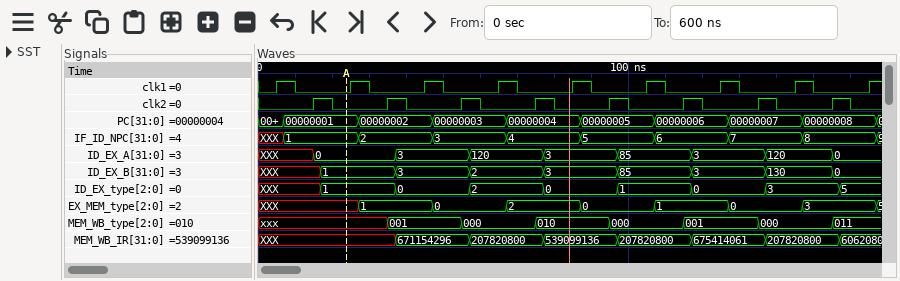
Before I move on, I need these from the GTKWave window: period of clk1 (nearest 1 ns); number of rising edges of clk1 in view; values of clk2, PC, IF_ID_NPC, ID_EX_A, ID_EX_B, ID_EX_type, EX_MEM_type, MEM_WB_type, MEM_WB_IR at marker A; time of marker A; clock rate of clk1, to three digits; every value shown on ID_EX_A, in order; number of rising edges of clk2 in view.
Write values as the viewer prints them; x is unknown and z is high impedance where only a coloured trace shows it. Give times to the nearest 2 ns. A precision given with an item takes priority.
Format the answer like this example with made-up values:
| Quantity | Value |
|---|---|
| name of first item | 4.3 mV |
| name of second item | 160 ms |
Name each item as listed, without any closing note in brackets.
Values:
| Quantity | Value |
|---|---|
| period of clk1 | 20 ns |
| number of rising edges of clk1 in view | 9 |
| values of clk2, PC, IF_ID_NPC, ID_EX_A, ID_EX_B, ID_EX_type, EX_MEM_type, MEM_WB_type, MEM_WB_IR at marker A | clk2=0, PC=00000001, IF_ID_NPC=1, ID_EX_A=0, ID_EX_B=1, ID_EX_type=1, EX_MEM_type=XXX, MEM_WB_type=xxx, MEM_WB_IR=XXX |
| time of marker A | 24 ns |
| clock rate of clk1, to three digits | 50.0 MHz |
| every value shown on ID_EX_A, in order | XXX, 0, 3, 120, 3, 85, 3, 120, 0 |
| number of rising edges of clk2 in view | 8 |
